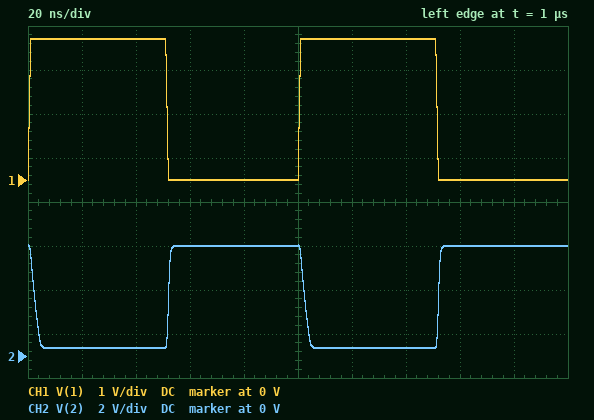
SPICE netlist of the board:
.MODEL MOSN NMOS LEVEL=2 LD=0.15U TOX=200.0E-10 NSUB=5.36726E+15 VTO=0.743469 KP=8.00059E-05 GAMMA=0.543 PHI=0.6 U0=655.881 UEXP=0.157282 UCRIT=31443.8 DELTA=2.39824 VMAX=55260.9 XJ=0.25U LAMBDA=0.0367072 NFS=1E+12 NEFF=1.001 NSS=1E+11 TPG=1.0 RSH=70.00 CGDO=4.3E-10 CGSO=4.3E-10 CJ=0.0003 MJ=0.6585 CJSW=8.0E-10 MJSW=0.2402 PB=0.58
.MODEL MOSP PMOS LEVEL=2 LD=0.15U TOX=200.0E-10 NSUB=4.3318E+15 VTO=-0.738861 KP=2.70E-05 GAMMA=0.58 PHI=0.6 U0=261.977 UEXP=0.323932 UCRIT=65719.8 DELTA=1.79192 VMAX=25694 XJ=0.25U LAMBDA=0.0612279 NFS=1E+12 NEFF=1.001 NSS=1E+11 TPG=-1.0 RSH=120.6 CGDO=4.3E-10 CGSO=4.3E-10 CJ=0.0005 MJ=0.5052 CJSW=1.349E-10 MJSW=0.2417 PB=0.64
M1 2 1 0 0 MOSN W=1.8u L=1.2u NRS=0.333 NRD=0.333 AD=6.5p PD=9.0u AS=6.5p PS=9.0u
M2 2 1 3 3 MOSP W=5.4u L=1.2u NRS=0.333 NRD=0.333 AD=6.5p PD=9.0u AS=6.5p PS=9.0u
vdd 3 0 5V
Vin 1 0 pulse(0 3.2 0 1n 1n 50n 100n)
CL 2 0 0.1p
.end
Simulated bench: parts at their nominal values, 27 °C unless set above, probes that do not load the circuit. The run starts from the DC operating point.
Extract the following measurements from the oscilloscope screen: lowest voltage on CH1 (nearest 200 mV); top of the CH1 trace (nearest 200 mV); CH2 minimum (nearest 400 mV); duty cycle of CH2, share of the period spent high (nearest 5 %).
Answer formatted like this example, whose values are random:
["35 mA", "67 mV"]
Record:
["0 V", "3.2 V", "400 mV", "50 %"]
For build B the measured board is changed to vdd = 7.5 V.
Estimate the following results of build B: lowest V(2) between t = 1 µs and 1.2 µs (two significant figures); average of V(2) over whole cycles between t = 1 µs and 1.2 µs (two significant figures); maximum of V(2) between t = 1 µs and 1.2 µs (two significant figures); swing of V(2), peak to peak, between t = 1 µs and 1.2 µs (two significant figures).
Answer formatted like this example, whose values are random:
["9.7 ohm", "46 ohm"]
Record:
["6.5 V", "7.0 V", "7.5 V", "1.0 V"]
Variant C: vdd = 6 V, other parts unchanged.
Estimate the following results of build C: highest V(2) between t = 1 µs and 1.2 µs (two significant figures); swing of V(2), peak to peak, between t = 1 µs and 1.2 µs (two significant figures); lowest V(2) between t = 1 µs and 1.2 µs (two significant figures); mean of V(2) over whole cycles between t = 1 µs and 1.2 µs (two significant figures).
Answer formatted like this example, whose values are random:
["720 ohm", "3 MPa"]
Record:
["6.0 V", "3.9 V", "2.2 V", "4.2 V"]
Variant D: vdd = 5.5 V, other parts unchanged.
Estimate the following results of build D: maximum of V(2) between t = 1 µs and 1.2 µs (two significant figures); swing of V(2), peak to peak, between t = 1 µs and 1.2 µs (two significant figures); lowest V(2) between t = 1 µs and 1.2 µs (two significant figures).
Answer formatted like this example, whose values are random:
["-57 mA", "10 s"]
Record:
["5.5 V", "4.9 V", "670 mV"]
